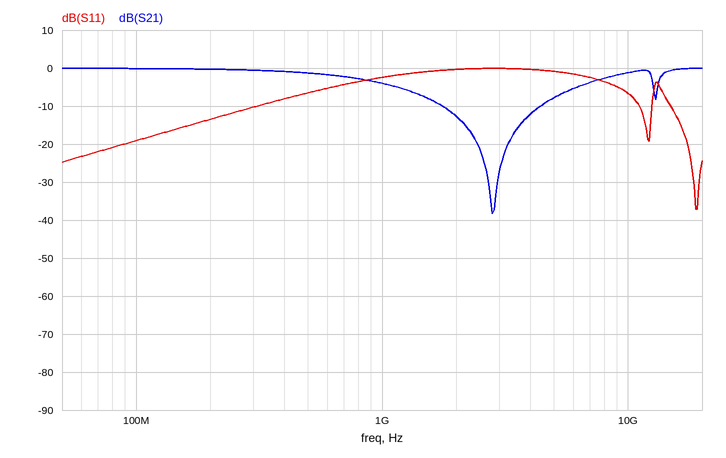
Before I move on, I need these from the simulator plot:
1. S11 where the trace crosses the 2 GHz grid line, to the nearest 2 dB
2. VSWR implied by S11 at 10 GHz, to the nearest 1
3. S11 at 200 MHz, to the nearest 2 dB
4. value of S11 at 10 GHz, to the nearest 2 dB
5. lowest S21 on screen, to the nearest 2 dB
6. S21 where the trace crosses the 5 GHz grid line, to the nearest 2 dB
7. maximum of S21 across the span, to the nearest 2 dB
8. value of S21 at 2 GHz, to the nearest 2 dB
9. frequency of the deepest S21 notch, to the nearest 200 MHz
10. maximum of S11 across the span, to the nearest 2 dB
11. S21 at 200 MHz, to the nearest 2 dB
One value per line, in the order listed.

0 dB
3
-14 dB
-6 dB
-38 dB
-8 dB
0 dB
-12 dB
2.8 GHz
0 dB
0 dB
